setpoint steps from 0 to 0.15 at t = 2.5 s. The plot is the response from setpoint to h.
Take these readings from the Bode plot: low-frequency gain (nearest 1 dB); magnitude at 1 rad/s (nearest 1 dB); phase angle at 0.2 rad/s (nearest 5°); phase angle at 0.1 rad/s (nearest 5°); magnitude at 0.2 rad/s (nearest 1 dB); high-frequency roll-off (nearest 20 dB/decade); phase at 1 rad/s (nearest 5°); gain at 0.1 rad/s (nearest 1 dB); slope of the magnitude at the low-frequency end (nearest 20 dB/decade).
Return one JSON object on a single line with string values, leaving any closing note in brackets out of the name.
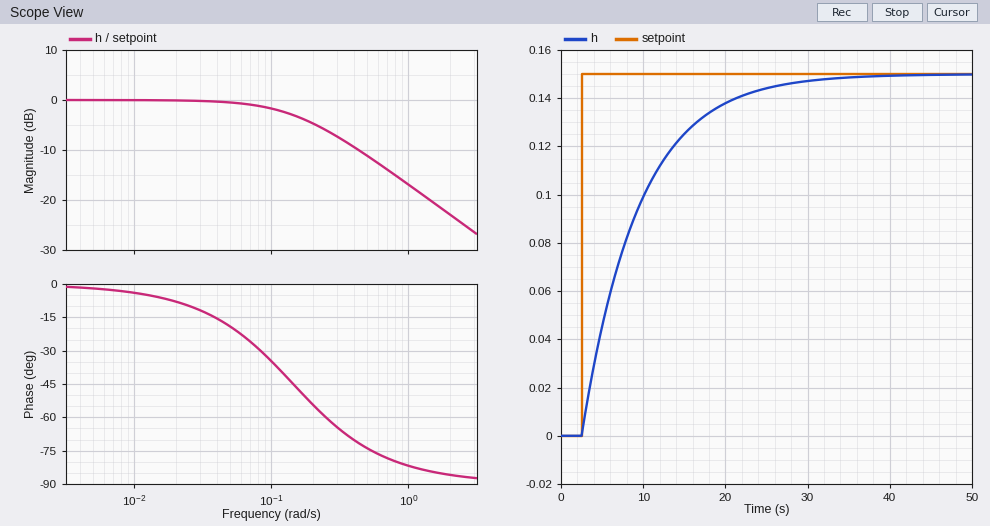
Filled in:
{"low-frequency gain": "0 dB", "magnitude at 1 rad/s": "-17 dB", "phase angle at 0.2 rad/s": "-55°", "phase angle at 0.1 rad/s": "-35°", "magnitude at 0.2 rad/s": "-5 dB", "high-frequency roll-off": "-20 dB/decade", "phase at 1 rad/s": "-80°", "gain at 0.1 rad/s": "-2 dB", "slope of the magnitude at the low-frequency end": "0 dB/decade"}
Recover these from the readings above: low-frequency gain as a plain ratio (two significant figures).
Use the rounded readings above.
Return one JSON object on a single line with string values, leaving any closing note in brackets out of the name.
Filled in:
{"low-frequency gain as a plain ratio": "1.0"}
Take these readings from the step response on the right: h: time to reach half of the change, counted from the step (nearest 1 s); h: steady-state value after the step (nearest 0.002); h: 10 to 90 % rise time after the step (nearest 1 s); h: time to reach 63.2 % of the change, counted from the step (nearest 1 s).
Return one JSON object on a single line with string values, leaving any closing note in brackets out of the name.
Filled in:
{"h: time to reach half of the change, counted from the step": "5 s", "h: steady-state value after the step": "0.150", "h: 10 to 90 % rise time after the step": "15 s", "h: time to reach 63.2 % of the change, counted from the step": "7 s"}
